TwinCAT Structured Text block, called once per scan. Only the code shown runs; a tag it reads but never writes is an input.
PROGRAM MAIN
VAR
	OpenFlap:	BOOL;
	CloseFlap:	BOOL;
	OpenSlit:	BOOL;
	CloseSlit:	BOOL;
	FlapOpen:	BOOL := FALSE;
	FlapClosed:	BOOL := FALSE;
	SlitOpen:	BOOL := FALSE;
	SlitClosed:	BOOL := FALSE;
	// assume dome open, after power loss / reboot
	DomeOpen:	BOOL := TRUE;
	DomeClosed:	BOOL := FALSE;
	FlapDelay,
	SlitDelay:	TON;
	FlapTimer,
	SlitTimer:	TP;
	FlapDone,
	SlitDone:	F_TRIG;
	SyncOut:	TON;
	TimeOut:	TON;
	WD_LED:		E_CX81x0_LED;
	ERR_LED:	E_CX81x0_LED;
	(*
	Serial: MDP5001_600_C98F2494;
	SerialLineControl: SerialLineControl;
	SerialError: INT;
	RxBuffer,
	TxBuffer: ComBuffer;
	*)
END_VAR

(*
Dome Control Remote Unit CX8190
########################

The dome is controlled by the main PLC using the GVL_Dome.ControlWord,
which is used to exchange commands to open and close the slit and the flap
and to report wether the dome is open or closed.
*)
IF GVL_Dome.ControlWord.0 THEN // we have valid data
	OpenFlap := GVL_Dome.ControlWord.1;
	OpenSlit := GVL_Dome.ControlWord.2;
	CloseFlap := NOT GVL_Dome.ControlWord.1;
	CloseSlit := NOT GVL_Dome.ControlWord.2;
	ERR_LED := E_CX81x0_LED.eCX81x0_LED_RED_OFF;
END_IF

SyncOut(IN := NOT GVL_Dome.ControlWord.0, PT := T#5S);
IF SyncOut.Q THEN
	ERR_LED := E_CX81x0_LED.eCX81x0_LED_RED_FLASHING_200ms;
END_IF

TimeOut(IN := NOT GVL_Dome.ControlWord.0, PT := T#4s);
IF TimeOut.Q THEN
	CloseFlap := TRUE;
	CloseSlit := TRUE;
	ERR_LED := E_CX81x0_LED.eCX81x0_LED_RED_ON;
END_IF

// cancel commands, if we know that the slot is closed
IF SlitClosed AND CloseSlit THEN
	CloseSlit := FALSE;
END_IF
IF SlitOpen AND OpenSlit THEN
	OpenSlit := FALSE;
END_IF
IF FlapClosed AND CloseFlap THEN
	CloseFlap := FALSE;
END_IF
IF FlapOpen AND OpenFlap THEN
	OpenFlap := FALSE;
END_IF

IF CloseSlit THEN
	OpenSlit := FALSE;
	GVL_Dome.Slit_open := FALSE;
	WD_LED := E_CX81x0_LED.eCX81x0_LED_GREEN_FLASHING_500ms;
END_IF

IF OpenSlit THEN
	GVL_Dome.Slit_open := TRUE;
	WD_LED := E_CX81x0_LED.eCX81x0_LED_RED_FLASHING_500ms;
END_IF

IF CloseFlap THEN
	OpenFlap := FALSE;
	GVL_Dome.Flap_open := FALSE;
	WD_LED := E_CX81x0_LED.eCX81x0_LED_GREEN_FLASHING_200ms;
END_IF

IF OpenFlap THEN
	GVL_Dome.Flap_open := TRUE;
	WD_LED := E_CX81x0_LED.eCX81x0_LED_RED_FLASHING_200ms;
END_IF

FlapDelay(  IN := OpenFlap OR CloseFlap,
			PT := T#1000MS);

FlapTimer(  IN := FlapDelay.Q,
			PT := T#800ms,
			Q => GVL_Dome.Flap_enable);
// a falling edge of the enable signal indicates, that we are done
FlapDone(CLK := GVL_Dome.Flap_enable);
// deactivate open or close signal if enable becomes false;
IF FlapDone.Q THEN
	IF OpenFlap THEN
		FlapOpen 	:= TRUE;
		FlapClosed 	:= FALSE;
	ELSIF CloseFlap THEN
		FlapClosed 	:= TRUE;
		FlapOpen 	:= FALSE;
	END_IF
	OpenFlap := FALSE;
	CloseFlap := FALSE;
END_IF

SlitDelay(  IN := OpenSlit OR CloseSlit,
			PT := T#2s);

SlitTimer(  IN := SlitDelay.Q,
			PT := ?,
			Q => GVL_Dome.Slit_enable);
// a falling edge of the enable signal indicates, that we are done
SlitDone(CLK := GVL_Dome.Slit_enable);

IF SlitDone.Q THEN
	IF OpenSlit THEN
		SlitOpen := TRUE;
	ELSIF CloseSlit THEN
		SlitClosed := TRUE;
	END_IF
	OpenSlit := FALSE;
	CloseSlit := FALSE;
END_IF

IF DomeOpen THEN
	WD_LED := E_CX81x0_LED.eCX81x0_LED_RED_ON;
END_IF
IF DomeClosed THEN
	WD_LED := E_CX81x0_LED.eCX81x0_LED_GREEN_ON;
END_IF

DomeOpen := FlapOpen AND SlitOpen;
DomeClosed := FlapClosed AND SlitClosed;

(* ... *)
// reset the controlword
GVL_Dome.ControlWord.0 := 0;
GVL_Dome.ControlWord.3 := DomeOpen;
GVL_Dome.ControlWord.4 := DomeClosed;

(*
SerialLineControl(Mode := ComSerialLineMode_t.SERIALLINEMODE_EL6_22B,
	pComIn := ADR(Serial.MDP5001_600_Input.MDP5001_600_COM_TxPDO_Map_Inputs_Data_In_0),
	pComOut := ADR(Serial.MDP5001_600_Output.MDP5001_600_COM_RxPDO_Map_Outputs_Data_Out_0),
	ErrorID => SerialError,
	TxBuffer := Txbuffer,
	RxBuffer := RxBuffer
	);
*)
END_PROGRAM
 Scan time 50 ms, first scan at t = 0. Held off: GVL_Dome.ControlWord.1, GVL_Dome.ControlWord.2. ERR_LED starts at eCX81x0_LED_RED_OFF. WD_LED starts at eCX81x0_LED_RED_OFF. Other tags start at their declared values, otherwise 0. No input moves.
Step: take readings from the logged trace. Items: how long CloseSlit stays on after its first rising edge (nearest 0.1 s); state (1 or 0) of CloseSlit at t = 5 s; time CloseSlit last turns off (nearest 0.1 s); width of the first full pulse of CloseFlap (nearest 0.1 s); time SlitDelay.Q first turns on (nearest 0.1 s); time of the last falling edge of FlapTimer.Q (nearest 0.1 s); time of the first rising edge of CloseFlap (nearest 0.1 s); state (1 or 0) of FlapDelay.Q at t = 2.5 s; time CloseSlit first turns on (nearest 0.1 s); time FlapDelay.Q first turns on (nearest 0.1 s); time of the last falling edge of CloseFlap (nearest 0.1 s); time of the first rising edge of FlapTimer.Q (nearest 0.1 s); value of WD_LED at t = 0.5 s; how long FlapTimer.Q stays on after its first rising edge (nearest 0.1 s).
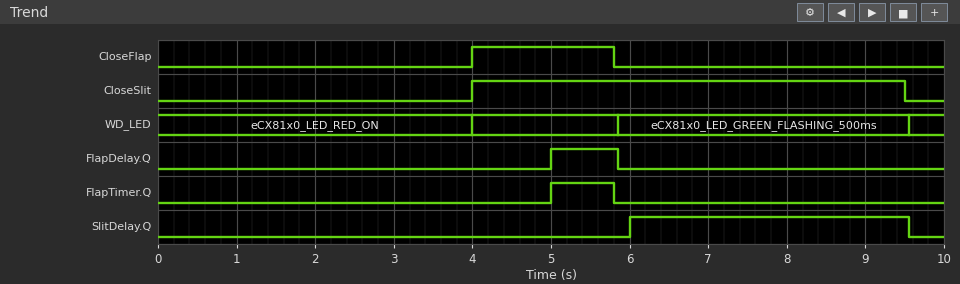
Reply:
5.5 s
1
9.5 s
1.8 s
6.0 s
5.8 s
4.0 s
0
4.0 s
5.0 s
5.8 s
5.0 s
eCX81x0_LED_RED_ON
0.8 s
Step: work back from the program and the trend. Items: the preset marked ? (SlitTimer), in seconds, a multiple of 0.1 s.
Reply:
3.5 s
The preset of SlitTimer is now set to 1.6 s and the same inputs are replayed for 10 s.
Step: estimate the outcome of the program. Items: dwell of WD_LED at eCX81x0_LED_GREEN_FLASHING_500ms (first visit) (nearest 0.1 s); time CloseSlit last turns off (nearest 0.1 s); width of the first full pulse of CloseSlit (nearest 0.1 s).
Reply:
1.8 s
7.6 s
3.6 s
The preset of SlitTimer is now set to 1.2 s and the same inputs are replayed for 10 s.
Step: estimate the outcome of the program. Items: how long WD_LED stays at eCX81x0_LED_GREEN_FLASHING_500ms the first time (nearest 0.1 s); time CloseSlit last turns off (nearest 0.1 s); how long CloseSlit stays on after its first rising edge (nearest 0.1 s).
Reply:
1.4 s
7.2 s
3.2 s
